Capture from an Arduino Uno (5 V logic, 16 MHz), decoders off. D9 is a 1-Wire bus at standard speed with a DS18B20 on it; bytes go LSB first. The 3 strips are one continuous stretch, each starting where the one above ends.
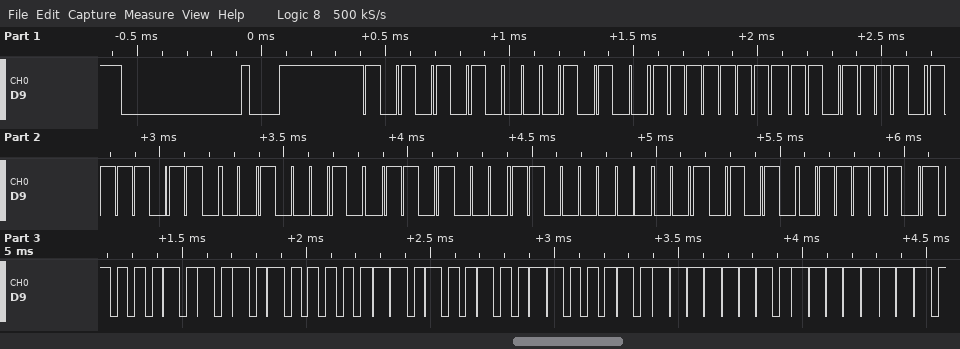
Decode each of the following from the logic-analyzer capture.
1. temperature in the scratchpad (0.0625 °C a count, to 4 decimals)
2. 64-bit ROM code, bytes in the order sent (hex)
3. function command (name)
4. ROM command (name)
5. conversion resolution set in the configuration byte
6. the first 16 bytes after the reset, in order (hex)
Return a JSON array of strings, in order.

["85.0000 °C", "28 FF 7B 6F 44 16 03 54", "Read Scratchpad", "Match ROM", "12 bits", "55 28 FF 7B 6F 44 16 03 54 BE 50 05 4B 46 7F FF"]
